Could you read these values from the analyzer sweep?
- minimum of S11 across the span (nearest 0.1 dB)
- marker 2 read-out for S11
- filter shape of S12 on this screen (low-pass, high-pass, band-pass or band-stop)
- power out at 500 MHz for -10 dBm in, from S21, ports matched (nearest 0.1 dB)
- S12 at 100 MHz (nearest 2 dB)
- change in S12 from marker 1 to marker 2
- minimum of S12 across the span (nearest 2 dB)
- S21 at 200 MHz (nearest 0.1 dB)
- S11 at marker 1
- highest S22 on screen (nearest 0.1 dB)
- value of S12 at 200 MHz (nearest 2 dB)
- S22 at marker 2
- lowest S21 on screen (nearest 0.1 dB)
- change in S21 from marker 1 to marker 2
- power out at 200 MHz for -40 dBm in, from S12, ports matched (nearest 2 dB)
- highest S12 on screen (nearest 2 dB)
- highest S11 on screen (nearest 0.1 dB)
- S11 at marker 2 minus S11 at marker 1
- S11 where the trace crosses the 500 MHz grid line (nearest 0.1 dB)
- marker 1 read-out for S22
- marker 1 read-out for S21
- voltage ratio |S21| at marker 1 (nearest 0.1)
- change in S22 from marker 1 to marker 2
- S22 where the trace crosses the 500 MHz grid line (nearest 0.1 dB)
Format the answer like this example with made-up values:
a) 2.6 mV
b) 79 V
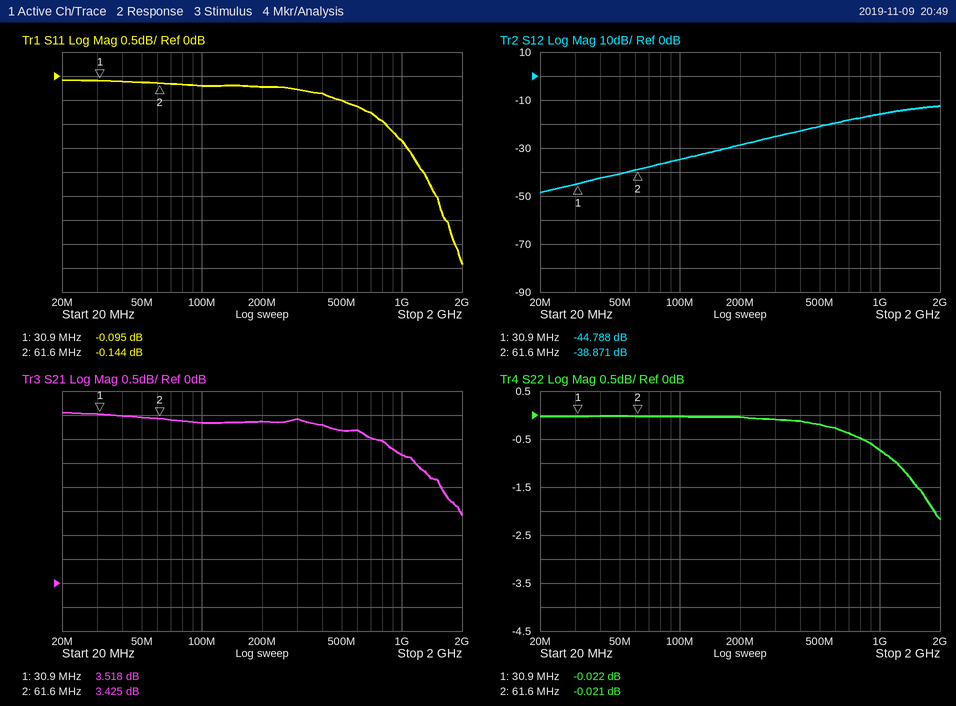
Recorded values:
a) -3.9 dB
b) -0.144 dB
c) high-pass
d) -6.8 dBm
e) -34 dB
f) 5.917 dB
g) -48 dB
h) 3.4 dB
i) -0.095 dB
j) 0.0 dB
k) -28 dB
l) -0.021 dB
m) 1.4 dB
n) -0.093 dB
o) -68 dBm
p) -12 dB
q) -0.1 dB
r) -0.049 dB
s) -0.5 dB
t) -0.022 dB
u) 3.518 dB
v) 1.5
w) 0.001 dB
x) -0.2 dB
